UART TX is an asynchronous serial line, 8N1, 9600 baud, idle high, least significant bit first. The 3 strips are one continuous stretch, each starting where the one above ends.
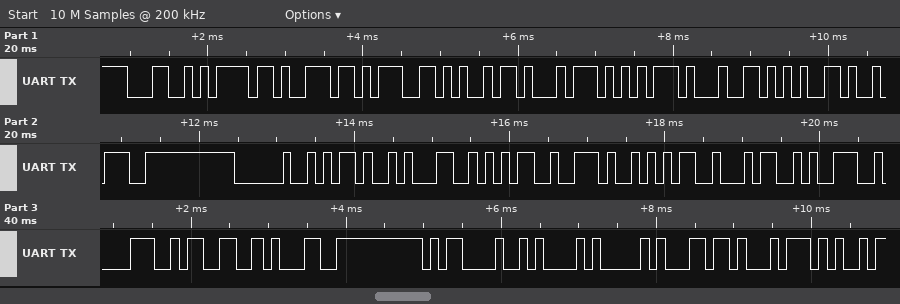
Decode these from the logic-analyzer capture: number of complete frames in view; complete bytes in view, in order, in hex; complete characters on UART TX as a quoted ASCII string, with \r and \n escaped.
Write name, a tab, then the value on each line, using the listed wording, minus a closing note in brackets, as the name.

number of complete frames in view	26
complete bytes in view, in order, in hex	0x4C 0x6F 0x6E 0x67 0x69 0x74 0x75 0x64 0x65 0x3A 0x20 0x2D 0x31 0x35 0x2E 0x35 0x34 0x39 0x38 0x33 0x31 0x0D 0x0A 0x41 0x6C 0x74
complete characters on UART TX as a quoted ASCII string, with \r and \n escaped	"Longitude: -15.549831\r\nAlt"
